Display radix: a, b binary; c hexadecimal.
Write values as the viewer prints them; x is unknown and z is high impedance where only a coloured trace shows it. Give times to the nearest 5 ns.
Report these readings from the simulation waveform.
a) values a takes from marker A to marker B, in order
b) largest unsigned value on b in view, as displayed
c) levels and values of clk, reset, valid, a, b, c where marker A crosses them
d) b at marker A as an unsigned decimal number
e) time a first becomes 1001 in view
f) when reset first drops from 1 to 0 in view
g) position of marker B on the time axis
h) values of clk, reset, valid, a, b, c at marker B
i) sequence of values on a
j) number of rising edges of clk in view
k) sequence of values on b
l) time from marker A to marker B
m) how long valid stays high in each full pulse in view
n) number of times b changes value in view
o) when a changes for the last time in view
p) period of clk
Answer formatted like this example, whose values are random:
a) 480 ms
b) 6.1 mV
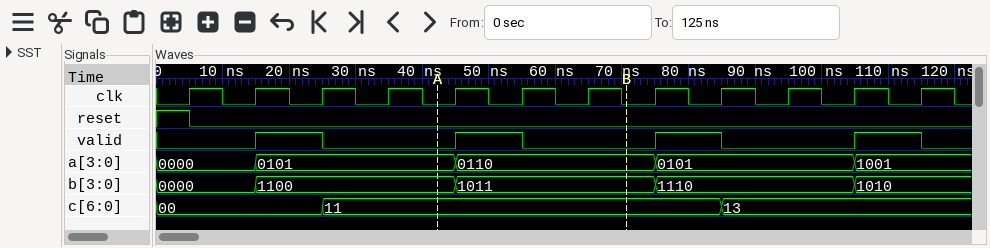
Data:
a) 0101, 0110
b) 1110
c) clk=0, reset=0, valid=0, a=0101, b=1100, c=11
d) 12
e) 105 ns
f) 5 ns
g) 70 ns
h) clk=0, reset=0, valid=0, a=0110, b=1011, c=11
i) 0000, 0101, 0110, 0101, 1001
j) 12
k) 0000, 1100, 1011, 1110, 1010
l) 30 ns
m) 10 ns, 10 ns, 10 ns, 10 ns
n) 4
o) 105 ns
p) 10 ns
